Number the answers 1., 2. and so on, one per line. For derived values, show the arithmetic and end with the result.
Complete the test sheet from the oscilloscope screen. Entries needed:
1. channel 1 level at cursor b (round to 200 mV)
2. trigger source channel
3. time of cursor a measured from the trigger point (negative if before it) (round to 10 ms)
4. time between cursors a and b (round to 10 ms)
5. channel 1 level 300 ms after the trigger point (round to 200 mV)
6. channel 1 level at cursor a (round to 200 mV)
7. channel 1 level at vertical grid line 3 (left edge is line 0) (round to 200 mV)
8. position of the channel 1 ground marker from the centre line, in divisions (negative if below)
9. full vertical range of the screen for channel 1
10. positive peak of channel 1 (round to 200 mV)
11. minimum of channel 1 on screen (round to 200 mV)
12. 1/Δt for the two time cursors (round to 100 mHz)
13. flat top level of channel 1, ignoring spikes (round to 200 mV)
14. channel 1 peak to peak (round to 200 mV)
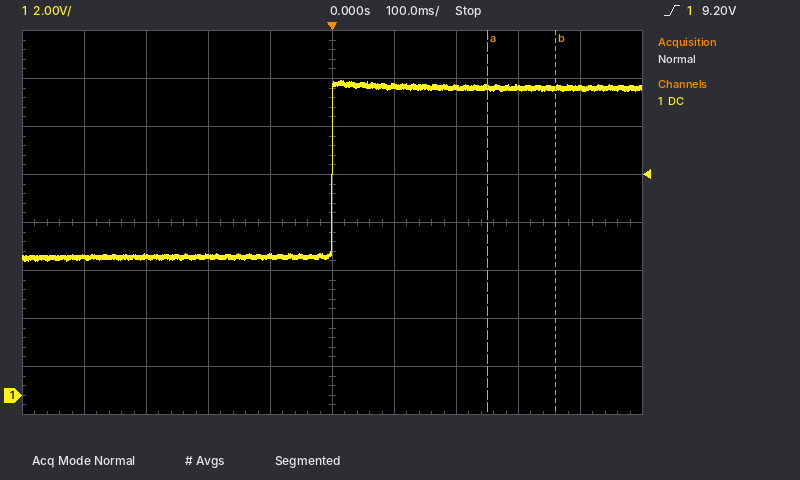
1. 12.8 V
2. channel 1
3. +250 ms
4. 110 ms
5. 12.8 V
6. 12.8 V
7. 5.8 V
8. -3.6 div
9. 16 V
10. 13.2 V
11. 5.6 V
12. 1 / 110 ms ≈ 9.1 Hz
13. 12.8 V
14. 13.2 V − (5.6 V) = 7.6 V
